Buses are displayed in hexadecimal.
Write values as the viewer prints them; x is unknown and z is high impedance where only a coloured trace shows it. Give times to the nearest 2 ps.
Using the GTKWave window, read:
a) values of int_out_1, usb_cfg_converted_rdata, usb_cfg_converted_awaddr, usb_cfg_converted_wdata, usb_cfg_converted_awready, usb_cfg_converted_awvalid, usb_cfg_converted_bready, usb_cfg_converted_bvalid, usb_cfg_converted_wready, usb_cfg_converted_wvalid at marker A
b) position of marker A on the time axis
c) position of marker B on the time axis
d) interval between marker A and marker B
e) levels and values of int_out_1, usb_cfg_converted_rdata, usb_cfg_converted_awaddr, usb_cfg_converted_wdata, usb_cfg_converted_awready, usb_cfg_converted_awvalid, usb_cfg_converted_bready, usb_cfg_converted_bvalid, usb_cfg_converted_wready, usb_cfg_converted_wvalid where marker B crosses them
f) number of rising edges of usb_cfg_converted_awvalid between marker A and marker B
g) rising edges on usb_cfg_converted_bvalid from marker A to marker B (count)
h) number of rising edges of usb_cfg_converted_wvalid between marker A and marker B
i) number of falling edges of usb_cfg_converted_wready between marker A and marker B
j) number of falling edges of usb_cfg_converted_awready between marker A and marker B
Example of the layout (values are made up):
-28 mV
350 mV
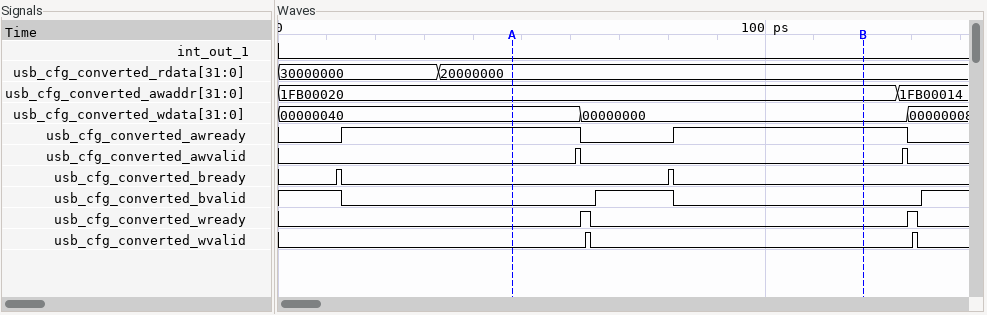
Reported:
int_out_1=0, usb_cfg_converted_rdata=20000000, usb_cfg_converted_awaddr=1FB00020, usb_cfg_converted_wdata=00000040, usb_cfg_converted_awready=1, usb_cfg_converted_awvalid=0, usb_cfg_converted_bready=0, usb_cfg_converted_bvalid=0, usb_cfg_converted_wready=0, usb_cfg_converted_wvalid=0
48 ps
120 ps
72 ps
int_out_1=0, usb_cfg_converted_rdata=20000000, usb_cfg_converted_awaddr=1FB00020, usb_cfg_converted_wdata=00000000, usb_cfg_converted_awready=1, usb_cfg_converted_awvalid=0, usb_cfg_converted_bready=0, usb_cfg_converted_bvalid=0, usb_cfg_converted_wready=0, usb_cfg_converted_wvalid=0
1
1
1
1
1
